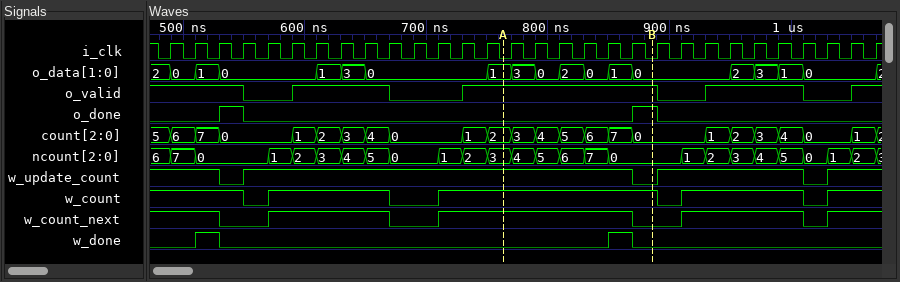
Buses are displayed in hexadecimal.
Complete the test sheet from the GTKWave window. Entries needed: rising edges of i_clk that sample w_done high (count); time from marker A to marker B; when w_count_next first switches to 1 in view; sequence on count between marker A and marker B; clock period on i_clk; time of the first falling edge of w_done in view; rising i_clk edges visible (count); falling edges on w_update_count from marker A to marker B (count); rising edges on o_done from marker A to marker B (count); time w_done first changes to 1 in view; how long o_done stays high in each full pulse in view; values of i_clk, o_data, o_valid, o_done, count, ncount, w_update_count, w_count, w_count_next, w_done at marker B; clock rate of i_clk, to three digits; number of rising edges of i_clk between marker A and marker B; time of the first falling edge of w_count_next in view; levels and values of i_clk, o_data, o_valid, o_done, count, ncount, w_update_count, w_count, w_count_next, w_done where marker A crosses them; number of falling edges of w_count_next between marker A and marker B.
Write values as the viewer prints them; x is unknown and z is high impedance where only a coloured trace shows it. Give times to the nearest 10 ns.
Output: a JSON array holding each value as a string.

["2", "120 ns", "570 ns", "2, 3, 4, 5, 6, 7, 0", "20 ns", "530 ns", "30", "1", "1", "510 ns", "20 ns, 20 ns", "i_clk=0, o_data=0, o_valid=1, o_done=1, count=0, ncount=0, w_update_count=0, w_count=1, w_count_next=0, w_done=0", "50.0 MHz", "6", "530 ns", "i_clk=0, o_data=1, o_valid=1, o_done=0, count=2, ncount=3, w_update_count=1, w_count=1, w_count_next=1, w_done=0", "1"]
